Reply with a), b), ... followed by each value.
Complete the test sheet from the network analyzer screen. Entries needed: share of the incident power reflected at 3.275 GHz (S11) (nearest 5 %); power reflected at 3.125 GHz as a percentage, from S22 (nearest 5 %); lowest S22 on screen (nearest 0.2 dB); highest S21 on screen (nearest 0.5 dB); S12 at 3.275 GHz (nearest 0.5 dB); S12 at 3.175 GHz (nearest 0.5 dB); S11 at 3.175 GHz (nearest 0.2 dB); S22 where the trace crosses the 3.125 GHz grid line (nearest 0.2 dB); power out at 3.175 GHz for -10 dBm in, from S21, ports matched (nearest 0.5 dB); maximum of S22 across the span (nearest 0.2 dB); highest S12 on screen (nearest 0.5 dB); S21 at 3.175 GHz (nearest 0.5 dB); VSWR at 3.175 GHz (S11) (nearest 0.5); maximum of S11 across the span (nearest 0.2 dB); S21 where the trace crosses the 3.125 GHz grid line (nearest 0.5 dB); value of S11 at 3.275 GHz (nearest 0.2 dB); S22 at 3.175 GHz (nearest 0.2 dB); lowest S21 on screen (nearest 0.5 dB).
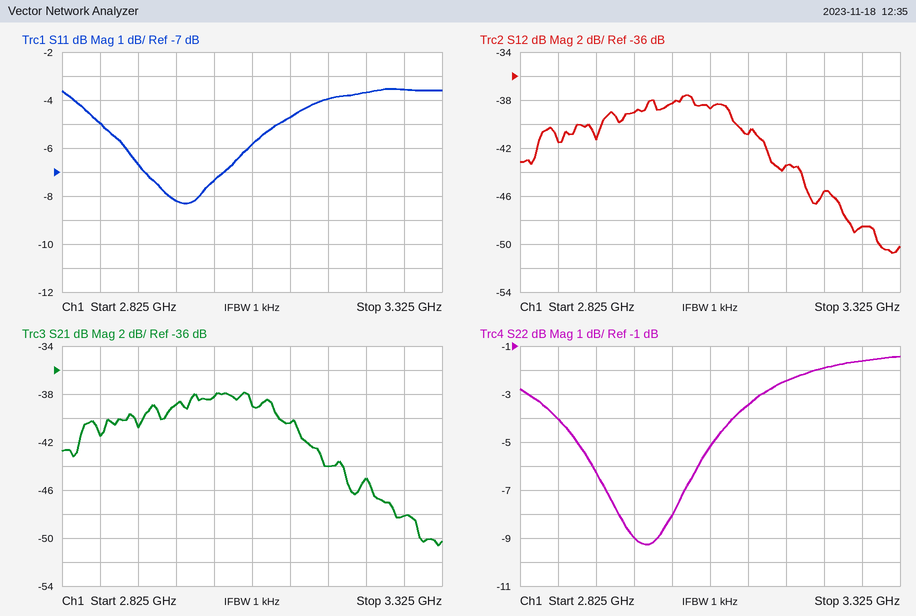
a) 45 %
b) 45 %
c) -9.2 dB
d) -38.0 dB
e) -48.5 dB
f) -43.5 dB
g) -4.0 dB
h) -3.4 dB
i) -54.0 dBm
j) -1.4 dB
k) -37.5 dB
l) -44.0 dB
m) 4.5
n) -3.6 dB
o) -40.5 dB
p) -3.6 dB
q) -2.4 dB
r) -50.5 dB
